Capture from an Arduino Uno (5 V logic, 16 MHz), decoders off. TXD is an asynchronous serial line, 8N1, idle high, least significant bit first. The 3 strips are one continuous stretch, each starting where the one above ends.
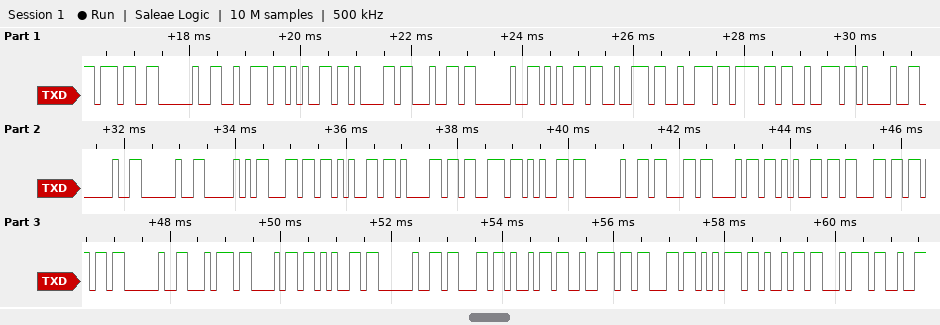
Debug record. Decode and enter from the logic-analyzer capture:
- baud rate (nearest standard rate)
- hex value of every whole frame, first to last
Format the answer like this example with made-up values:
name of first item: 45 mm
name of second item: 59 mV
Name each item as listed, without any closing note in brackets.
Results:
baud rate: 9600 baud
hex value of every whole frame, first to last: 0x37 0x20 0x72 0x65 0x61 0x64 0x20 0x65 0x72 0x72 0x6F 0x72 0x21 0x20 0x20 0x50 0x6C 0x65 0x61 0x73 0x65 0x20 0x63 0x68 0x65 0x63 0x6B 0x20 0x74 0x68 0x65 0x20 0x63 0x69 0x72 0x63 0x75 0x69 0x74
